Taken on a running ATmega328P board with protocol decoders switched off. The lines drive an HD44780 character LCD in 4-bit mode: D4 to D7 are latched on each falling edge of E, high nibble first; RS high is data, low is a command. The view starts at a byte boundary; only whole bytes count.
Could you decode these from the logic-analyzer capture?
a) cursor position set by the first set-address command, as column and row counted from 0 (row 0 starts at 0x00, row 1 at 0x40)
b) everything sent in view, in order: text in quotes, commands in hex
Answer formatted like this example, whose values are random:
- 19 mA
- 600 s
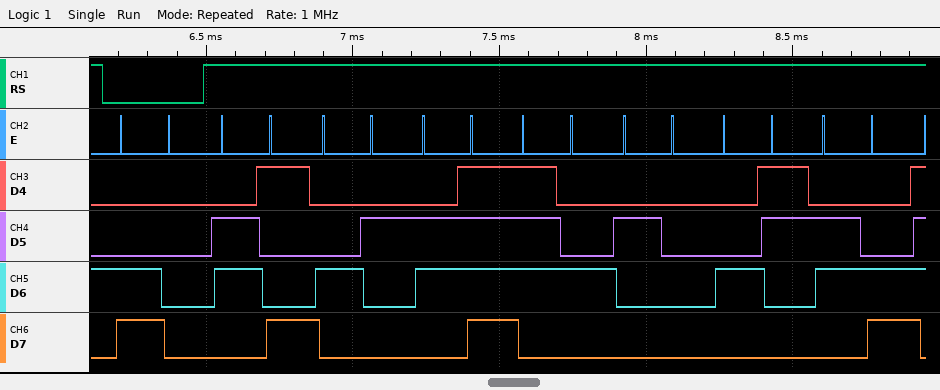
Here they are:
- column 0, row 1
- 0xC0 "iBot Cl"
